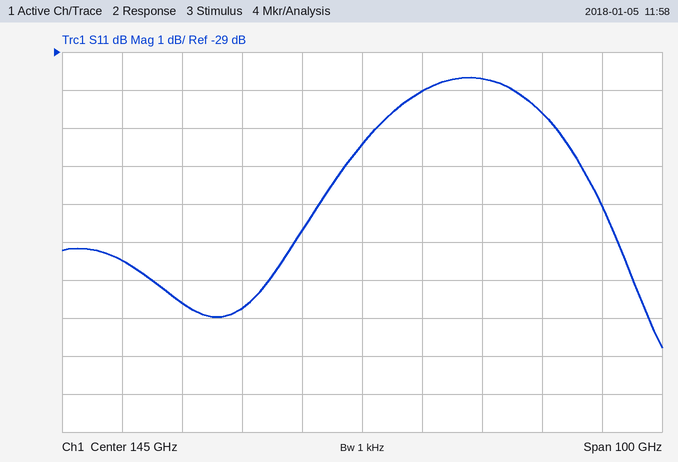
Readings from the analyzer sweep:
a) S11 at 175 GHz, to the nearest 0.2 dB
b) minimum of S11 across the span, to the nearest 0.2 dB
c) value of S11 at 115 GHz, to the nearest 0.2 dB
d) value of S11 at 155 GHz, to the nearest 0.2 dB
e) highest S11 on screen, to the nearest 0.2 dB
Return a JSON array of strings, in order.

["-30.6 dB", "-36.8 dB", "-35.6 dB", "-30.0 dB", "-29.6 dB"]
